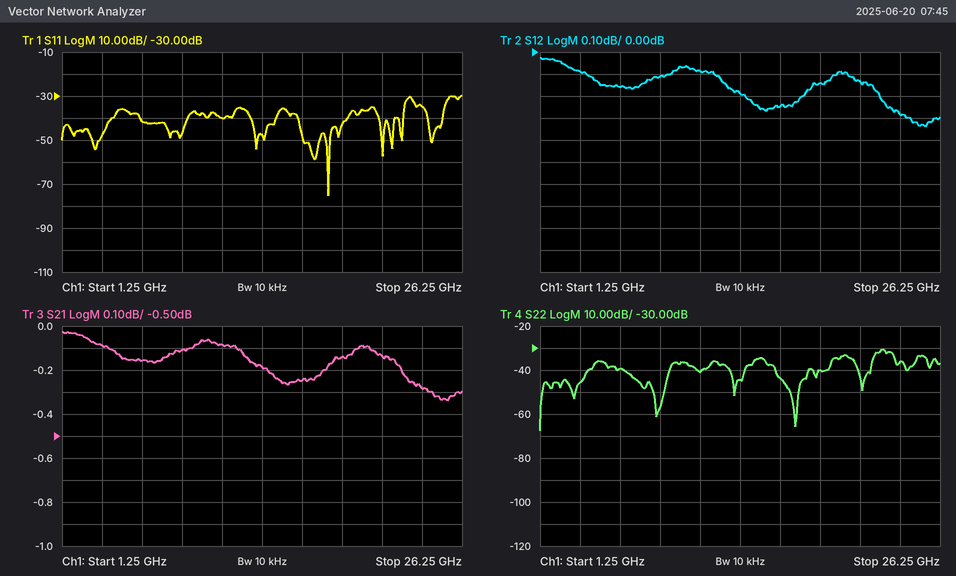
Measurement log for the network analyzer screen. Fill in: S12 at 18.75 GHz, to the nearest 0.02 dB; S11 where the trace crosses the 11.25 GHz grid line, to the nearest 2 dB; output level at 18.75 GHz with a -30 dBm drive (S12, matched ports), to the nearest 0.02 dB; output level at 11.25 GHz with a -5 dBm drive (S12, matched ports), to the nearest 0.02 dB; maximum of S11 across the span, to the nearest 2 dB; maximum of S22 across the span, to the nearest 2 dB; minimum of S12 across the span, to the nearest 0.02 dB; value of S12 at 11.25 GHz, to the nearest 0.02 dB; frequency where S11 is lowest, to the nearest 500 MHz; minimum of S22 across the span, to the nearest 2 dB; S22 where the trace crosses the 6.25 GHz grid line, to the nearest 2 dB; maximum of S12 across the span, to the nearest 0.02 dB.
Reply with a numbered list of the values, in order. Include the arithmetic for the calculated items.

1. -0.14 dB
2. -40 dB
3. -30 dBm + (-0.14 dB) = -30.14 dBm
4. -5 dBm + (-0.08 dB) = -5.08 dBm
5. -30 dB
6. -30 dB
7. -0.34 dB
8. -0.08 dB
9. 18.0 GHz
10. -68 dB
11. -40 dB
12. -0.02 dB
